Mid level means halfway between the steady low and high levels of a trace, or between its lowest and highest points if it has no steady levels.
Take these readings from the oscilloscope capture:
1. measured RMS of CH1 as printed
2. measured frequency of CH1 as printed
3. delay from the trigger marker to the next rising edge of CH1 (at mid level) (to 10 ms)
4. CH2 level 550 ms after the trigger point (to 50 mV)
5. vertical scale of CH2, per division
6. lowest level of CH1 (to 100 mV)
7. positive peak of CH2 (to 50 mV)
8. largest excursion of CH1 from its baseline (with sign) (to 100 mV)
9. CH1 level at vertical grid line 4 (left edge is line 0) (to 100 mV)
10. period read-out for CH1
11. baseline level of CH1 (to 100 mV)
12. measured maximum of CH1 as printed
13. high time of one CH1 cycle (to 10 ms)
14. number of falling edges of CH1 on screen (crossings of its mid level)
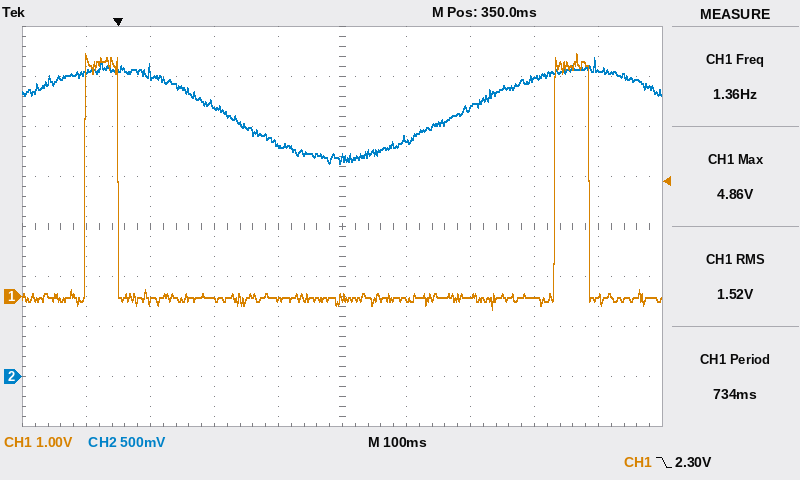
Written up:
1.52 V
1.36 Hz
680 ms
2.70 V
500 mV
-300 mV
3.20 V
+4.9 V
-100 mV
734 ms
0.0 V
4.86 V
50 ms
2
